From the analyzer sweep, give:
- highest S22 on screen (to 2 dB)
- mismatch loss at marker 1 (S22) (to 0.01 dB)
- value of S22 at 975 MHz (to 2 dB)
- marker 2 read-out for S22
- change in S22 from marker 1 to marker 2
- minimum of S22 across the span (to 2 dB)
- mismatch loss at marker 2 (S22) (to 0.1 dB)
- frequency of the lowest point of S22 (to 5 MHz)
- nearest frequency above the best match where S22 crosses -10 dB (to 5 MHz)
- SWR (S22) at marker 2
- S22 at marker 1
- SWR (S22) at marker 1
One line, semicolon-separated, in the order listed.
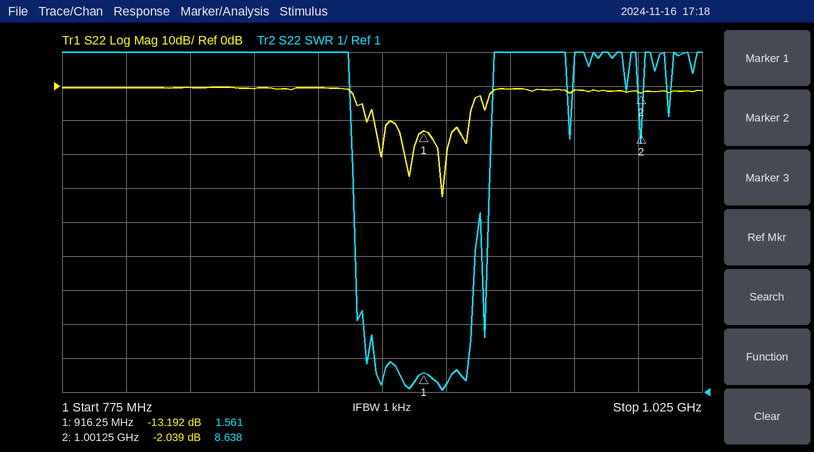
0 dB; 0.21 dB; -2 dB; -2.039 dB; 11.153 dB; -32 dB; 4.3 dB; 925 MHz; 935 MHz; 8.638; -13.192 dB; 1.561
